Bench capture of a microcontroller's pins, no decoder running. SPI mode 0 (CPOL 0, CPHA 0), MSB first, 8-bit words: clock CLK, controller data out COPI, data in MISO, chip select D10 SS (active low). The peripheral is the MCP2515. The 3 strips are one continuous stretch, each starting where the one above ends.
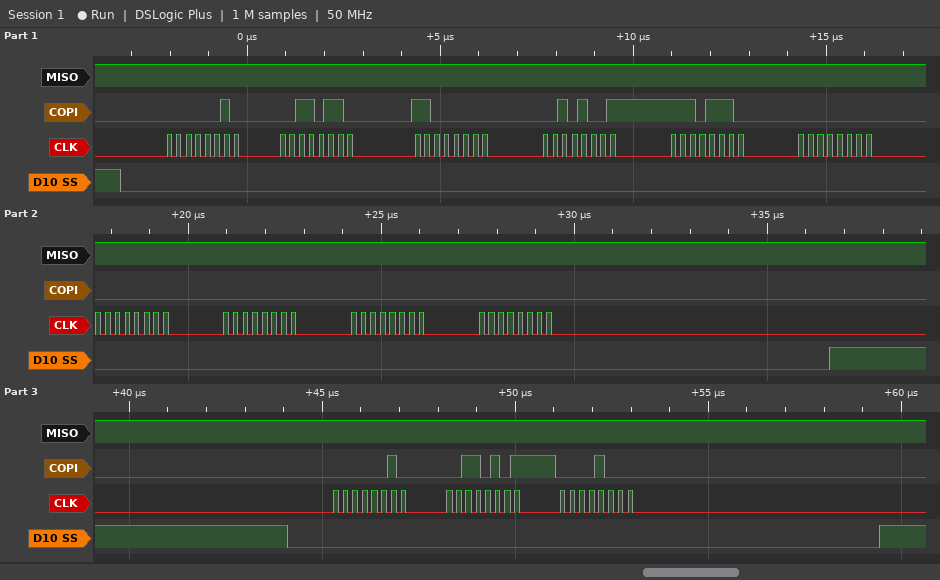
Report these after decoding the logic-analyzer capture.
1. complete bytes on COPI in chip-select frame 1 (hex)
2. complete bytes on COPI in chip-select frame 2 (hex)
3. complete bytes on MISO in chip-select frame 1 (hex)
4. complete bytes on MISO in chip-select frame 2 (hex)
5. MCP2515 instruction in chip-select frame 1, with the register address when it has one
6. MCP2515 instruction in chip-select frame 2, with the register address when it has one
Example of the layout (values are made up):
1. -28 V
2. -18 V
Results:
1. 02 36 C0 29 EE 00 00 00 00 00
2. 02 35 08
3. FF FF FF FF FF FF FF FF FF FF
4. FF FF FF
5. WRITE 0x36
6. WRITE 0x35
